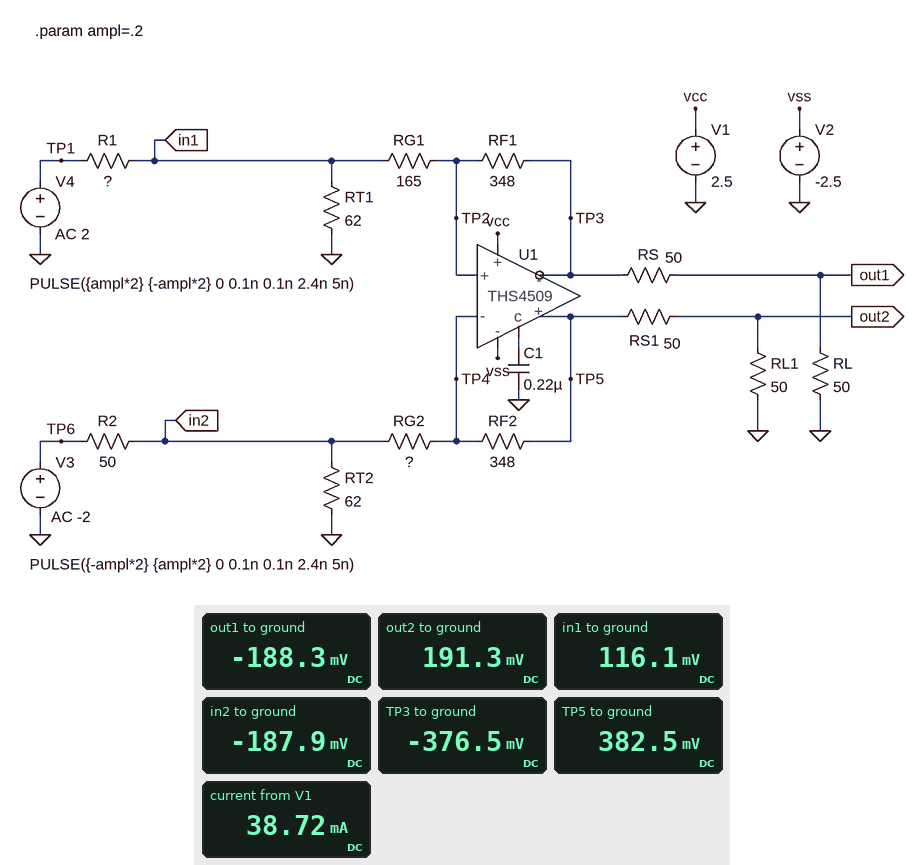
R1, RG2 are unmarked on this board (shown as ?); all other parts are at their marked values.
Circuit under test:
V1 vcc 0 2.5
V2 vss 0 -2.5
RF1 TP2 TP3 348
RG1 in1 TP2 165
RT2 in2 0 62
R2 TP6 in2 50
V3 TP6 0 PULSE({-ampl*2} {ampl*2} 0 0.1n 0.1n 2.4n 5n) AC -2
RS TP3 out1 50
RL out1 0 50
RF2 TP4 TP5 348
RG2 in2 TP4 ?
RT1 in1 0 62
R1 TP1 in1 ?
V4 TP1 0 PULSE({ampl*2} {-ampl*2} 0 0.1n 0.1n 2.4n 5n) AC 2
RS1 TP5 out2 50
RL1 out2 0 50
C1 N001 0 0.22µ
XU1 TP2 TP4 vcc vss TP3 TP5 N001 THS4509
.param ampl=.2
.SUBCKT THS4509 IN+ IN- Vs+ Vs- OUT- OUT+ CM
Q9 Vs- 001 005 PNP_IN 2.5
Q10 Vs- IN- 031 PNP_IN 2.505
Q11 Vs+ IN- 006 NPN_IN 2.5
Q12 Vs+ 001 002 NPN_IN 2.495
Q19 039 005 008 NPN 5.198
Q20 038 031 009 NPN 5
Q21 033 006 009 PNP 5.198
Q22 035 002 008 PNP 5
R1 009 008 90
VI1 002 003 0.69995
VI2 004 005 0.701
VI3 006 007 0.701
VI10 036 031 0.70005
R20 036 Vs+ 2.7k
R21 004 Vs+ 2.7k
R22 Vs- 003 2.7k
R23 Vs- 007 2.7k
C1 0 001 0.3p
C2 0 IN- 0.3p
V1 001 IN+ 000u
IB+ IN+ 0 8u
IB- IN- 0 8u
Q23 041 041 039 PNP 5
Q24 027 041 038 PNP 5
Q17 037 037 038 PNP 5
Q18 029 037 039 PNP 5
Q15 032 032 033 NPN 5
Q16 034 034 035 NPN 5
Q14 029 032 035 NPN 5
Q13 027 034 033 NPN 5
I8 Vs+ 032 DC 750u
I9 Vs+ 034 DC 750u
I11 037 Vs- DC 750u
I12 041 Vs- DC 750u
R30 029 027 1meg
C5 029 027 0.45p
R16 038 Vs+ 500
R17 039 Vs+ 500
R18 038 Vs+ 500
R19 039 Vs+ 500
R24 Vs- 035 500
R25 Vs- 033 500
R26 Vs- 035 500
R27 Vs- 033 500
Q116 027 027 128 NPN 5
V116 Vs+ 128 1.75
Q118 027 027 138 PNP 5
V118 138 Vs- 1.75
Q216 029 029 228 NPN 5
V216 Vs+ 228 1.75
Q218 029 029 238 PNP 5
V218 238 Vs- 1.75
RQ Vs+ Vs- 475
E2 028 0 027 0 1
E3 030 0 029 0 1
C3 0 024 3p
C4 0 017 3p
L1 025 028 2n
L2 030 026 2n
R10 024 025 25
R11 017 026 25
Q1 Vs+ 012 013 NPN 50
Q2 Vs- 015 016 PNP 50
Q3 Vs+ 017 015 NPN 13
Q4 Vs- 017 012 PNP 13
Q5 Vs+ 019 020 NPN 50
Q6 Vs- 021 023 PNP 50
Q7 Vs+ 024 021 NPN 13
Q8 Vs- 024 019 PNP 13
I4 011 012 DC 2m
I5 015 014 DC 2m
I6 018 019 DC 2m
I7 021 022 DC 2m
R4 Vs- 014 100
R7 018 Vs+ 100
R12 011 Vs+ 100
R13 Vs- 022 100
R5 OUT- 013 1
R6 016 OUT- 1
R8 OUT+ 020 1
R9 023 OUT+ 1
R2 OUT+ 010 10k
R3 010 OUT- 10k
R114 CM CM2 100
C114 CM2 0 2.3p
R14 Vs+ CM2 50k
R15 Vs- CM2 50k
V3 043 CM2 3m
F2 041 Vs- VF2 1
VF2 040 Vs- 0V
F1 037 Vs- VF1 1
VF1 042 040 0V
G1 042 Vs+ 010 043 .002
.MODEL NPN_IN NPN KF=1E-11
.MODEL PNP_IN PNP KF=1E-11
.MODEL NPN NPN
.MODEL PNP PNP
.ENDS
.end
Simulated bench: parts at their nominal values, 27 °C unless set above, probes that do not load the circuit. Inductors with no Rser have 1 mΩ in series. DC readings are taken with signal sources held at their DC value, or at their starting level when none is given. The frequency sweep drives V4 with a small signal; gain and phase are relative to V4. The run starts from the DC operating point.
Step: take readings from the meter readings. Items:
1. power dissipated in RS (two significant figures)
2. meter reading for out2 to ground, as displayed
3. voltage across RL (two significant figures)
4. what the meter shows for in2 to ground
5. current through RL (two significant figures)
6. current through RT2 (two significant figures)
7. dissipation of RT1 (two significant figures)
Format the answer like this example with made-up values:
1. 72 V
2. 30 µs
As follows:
1. 710 µW
2. 191.3 mV
3. 190 mV
4. -187.9 mV
5. 3.8 mA
6. 3.0 mA
7. 220 µW
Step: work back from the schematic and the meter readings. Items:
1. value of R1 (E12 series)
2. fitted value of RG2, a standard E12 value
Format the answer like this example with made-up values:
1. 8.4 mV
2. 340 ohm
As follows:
1. 100 Ω
2. 120 Ω
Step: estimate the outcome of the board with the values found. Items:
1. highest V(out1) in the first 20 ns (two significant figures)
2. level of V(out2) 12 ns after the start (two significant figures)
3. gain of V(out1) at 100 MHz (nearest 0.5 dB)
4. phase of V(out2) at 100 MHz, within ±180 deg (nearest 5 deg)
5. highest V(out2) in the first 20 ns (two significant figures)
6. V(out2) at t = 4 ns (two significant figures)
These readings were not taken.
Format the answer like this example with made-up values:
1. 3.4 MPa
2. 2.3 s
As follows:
1. 300 mV
2. -190 mV
3. -2.5 dB
4. -5 deg
5. 300 mV
6. 180 mV
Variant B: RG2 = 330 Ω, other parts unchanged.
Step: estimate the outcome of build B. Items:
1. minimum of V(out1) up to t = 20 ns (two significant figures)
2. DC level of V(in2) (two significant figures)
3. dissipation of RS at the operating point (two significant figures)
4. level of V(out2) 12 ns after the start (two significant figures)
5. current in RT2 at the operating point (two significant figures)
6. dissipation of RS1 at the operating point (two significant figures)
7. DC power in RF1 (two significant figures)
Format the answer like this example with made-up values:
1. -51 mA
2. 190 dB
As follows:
1. -240 mV
2. -200 mV
3. 270 µW
4. -110 mV
5. 3.3 mA
6. 290 µW
7. 170 µW
